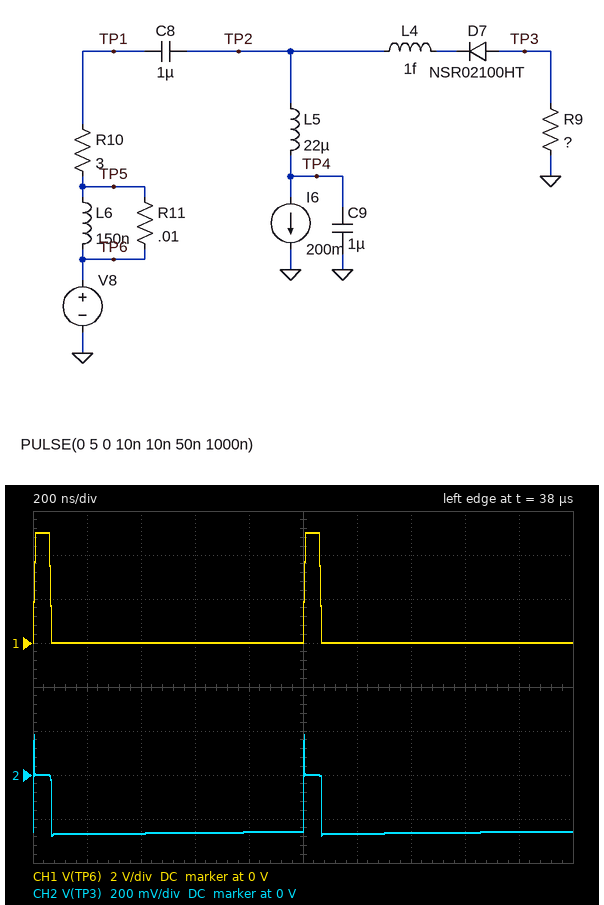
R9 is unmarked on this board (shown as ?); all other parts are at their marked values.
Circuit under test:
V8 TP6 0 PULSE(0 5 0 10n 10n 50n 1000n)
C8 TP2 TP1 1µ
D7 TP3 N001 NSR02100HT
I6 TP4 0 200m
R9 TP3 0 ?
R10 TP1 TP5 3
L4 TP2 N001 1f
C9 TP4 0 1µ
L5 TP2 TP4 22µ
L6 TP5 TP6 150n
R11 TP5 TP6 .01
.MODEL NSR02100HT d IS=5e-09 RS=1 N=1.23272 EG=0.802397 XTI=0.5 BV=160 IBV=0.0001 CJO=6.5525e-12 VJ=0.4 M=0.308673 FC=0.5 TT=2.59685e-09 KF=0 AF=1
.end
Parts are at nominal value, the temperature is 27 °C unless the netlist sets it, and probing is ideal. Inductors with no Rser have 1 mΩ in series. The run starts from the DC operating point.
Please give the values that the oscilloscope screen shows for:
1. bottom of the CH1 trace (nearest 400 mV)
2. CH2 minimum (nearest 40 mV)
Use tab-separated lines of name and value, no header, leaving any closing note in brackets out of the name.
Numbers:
bottom of the CH1 trace	0 V
CH2 minimum	-280 mV
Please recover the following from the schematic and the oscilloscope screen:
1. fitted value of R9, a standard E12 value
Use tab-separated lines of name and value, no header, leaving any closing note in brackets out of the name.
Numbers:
fitted value of R9, a standard E12 value	1.2 Ω
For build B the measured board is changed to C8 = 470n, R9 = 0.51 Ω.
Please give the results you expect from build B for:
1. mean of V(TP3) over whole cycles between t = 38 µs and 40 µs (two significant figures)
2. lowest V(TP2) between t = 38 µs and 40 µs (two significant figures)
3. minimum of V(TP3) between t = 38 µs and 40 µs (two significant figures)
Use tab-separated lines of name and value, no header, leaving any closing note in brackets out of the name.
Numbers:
mean of V(TP3) over whole cycles between t = 38 µs and 40 µs	-110 mV
lowest V(TP2) between t = 38 µs and 40 µs	-910 mV
minimum of V(TP3) between t = 38 µs and 40 µs	-120 mV
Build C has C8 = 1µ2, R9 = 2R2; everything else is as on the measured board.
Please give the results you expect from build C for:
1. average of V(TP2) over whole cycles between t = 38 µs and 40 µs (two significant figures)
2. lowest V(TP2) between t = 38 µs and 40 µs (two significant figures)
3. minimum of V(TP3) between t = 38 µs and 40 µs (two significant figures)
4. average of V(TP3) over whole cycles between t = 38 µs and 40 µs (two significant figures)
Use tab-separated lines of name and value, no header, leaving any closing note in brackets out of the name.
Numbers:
average of V(TP2) over whole cycles between t = 38 µs and 40 µs	-1.0 V
lowest V(TP2) between t = 38 µs and 40 µs	-1.3 V
minimum of V(TP3) between t = 38 µs and 40 µs	-500 mV
average of V(TP3) over whole cycles between t = 38 µs and 40 µs	-450 mV
